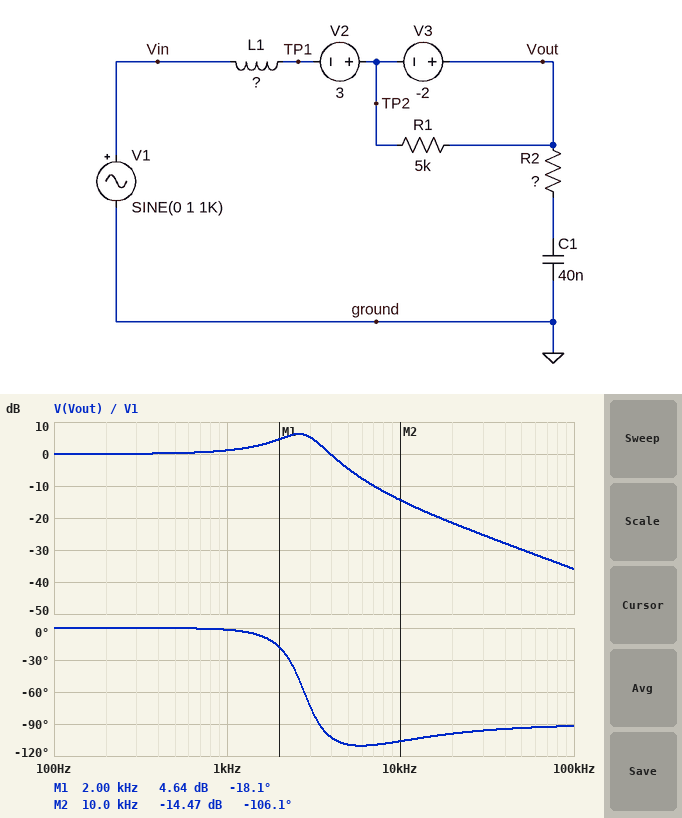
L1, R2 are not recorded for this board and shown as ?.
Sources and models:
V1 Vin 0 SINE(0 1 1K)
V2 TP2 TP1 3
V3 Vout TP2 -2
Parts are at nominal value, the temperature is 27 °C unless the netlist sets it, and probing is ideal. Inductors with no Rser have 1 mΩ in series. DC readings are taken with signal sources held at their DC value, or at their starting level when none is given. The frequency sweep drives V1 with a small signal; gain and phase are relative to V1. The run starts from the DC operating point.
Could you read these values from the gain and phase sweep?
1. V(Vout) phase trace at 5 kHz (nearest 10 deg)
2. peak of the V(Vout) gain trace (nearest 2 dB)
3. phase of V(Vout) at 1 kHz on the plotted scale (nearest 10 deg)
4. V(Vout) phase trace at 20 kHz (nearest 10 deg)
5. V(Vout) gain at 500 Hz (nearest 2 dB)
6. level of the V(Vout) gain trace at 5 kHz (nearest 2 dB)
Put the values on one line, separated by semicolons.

-110 deg; 6 dB; 0 deg; -100 deg; 0 dB; -4 dB
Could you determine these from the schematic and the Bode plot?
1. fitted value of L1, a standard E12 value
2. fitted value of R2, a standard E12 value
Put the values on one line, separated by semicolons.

82 mH; 820 Ω
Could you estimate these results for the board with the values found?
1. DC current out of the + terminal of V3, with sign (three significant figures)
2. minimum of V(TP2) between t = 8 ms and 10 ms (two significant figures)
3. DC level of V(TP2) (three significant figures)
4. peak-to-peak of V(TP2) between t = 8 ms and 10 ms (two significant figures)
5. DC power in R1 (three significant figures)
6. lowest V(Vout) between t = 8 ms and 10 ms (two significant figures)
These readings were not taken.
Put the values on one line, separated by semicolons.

-400 µA; 1.9 V; 3.00 V; 2.3 V; 800 µW; -140 mV
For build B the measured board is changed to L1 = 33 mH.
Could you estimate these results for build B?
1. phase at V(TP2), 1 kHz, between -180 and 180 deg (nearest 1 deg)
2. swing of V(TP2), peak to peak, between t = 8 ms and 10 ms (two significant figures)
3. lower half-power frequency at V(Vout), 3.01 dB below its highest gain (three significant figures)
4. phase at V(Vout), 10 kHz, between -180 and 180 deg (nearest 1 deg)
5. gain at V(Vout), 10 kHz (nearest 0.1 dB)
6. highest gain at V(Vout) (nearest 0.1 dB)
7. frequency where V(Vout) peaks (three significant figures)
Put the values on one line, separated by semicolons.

-1 deg; 2.1 V; 1.33 kHz; -90 deg; -6.2 dB; 3.8 dB; 3.83 kHz
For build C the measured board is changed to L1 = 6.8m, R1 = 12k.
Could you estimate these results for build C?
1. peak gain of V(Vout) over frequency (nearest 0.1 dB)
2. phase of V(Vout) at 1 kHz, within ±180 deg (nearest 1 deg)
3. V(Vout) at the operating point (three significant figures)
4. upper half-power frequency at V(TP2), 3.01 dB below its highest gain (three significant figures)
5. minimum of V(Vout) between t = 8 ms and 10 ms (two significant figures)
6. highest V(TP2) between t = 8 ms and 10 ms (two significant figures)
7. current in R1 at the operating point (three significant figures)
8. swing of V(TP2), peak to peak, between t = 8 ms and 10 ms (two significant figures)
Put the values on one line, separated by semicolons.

1.3 dB; 0 deg; 1.00 V; 19.5 kHz; -10 mV; 4.0 V; 167 µA; 2.0 V
